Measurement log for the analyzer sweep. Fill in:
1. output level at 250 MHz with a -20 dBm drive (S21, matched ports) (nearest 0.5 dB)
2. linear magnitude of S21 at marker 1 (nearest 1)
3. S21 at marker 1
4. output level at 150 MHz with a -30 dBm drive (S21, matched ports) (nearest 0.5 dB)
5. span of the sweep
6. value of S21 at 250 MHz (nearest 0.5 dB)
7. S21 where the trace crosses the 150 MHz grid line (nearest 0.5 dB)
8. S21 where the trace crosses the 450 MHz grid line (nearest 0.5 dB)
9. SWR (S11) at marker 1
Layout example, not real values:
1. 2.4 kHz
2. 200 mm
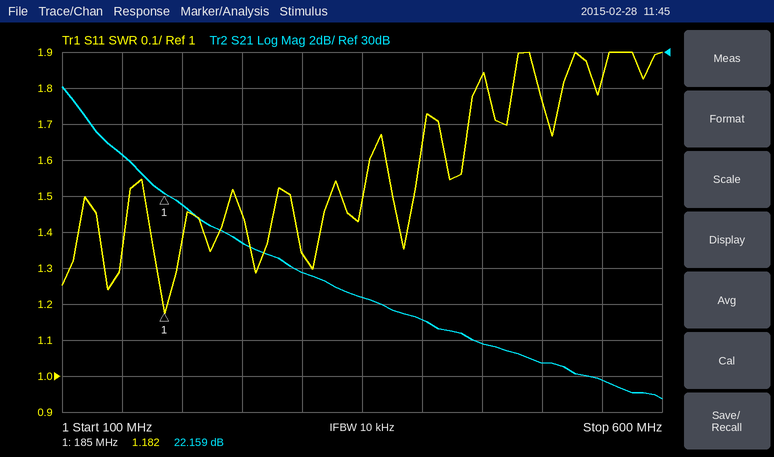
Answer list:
1. -0.5 dBm
2. 13
3. 22.159 dB
4. -5.5 dBm
5. 500 MHz
6. 19.5 dB
7. 24.5 dB
8. 14.0 dB
9. 1.182
